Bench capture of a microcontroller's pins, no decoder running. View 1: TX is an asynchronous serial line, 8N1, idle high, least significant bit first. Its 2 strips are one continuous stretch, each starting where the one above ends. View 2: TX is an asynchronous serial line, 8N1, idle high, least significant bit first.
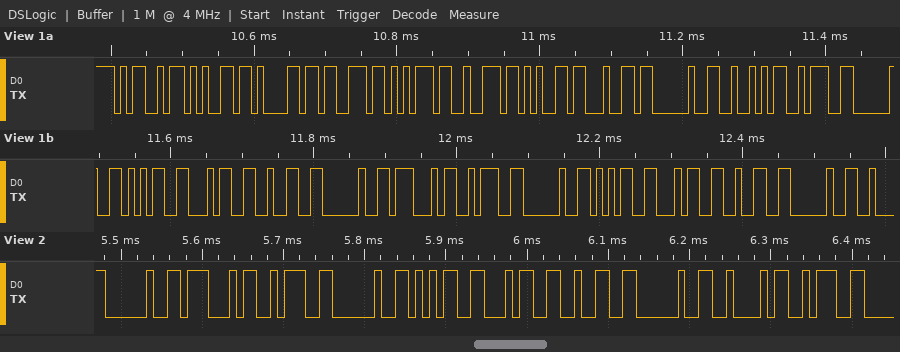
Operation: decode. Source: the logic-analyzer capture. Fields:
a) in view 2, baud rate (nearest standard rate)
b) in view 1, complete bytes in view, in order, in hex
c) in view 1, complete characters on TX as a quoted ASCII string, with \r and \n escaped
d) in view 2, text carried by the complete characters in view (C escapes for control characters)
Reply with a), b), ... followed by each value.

a) 115200 baud
b) 4D 65 61 73 75 72 65 64 20 52 3A 20 35 34 32 20 47 3A 20 35 34 32 20
c) "Measured R: 542 G: 542 "
d) " G: 542 B:"
